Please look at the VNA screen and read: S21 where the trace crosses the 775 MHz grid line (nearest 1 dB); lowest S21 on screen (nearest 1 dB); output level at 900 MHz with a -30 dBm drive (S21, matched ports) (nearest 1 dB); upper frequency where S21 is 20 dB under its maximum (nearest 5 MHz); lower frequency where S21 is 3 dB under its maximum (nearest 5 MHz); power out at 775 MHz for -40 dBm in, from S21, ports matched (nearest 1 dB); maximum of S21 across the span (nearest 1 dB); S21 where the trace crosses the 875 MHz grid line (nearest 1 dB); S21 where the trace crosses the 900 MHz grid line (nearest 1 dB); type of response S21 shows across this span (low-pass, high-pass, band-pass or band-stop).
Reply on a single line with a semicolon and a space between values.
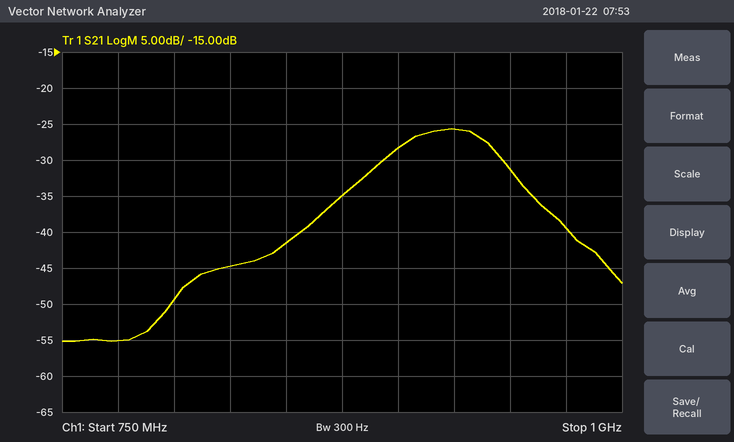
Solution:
-55 dB; -55 dB; -58 dBm; 995 MHz; 900 MHz; -95 dBm; -26 dB; -35 dB; -28 dB; band-pass
